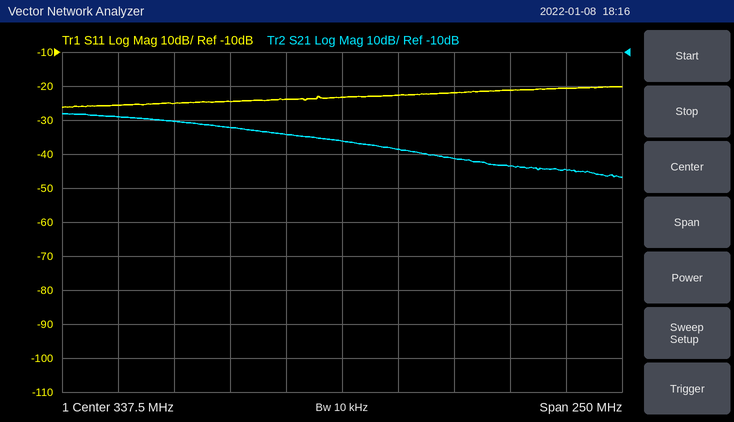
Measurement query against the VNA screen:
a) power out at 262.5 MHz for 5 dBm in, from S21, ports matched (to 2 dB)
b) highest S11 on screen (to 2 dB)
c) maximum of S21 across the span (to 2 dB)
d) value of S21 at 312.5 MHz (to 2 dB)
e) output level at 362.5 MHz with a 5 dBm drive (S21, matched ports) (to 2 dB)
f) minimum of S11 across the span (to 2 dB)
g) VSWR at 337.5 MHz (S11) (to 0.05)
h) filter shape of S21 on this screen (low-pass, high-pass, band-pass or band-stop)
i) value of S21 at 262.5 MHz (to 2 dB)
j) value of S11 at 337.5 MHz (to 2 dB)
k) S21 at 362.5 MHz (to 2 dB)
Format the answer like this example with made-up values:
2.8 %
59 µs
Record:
-26 dBm
-20 dB
-28 dB
-34 dB
-34 dBm
-26 dB
1.15
low-pass
-30 dB
-24 dB
-38 dB
